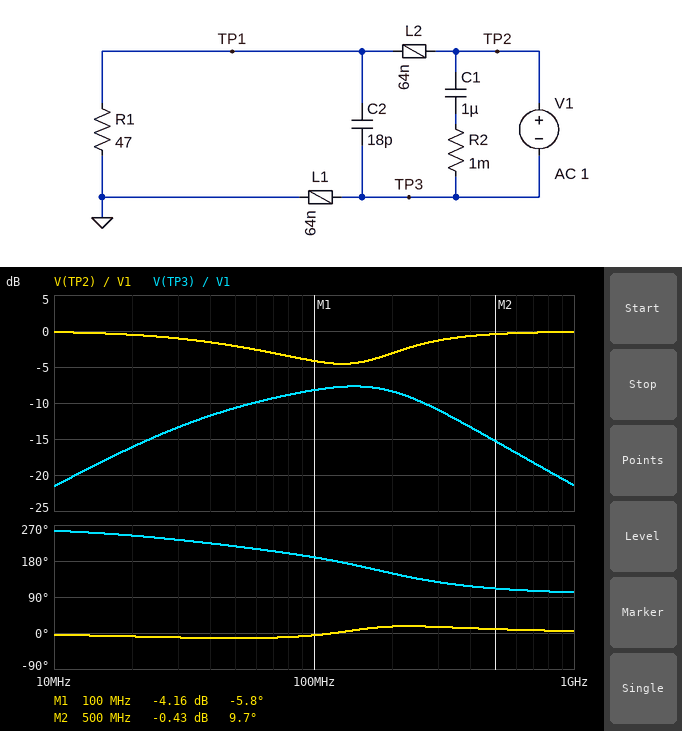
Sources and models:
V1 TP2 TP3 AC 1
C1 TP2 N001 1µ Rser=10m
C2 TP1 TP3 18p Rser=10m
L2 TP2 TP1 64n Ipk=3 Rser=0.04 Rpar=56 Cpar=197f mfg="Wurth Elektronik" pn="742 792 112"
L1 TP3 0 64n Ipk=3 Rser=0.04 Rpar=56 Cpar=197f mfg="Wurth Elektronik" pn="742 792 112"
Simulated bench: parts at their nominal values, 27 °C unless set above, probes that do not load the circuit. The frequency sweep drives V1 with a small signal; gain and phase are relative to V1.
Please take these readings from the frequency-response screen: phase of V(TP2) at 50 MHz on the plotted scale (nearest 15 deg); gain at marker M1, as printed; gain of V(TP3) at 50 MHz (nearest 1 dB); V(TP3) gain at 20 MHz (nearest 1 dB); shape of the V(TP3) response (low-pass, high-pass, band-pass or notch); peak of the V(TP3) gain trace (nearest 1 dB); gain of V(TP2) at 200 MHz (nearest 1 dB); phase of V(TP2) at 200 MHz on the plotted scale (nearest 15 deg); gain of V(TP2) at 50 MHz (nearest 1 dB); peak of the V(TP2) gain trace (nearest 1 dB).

-15 deg
-4.16 dB
-11 dB
-16 dB
band-pass
-8 dB
-3 dB
15 deg
-2 dB
0 dB
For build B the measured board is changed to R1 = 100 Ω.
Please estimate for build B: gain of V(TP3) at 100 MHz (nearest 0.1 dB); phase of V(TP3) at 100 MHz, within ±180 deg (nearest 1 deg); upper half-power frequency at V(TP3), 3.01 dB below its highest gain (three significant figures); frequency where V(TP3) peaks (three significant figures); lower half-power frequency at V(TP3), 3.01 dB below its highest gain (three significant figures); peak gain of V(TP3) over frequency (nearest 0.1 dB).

-11.3 dB
-162 deg
272 MHz
142 MHz
64.5 MHz
-10.5 dB
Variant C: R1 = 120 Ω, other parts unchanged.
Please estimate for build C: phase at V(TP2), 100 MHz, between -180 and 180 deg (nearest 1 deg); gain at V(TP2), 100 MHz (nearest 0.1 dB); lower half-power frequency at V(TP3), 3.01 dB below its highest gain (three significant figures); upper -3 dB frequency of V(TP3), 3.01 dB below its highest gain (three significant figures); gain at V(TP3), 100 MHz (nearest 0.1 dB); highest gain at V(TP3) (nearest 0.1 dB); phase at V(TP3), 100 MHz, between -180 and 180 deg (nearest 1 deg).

-6 deg
-2.2 dB
67.5 MHz
269 MHz
-12.2 dB
-11.4 dB
-160 deg
